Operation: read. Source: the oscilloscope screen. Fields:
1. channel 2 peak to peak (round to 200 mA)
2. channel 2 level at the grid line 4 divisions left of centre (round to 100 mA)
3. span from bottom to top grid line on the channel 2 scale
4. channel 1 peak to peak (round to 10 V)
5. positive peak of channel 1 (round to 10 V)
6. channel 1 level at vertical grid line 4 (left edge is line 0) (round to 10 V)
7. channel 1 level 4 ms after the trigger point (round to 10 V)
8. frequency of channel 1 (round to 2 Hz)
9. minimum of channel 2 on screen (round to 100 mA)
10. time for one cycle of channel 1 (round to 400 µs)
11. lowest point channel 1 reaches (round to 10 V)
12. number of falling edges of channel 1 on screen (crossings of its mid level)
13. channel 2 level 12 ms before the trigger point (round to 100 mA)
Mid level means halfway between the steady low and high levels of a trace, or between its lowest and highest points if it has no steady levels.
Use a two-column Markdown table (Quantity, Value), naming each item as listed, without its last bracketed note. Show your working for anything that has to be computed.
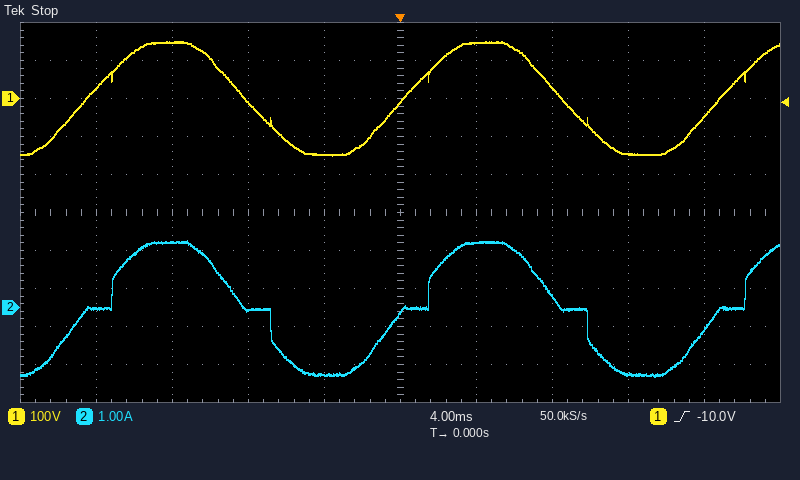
| Quantity | Value |
|---|---|
| channel 2 peak to peak | 3.6 A |
| channel 2 level at the grid line 4 divisions left of centre | 0.0 A |
| span from bottom to top grid line on the channel 2 scale | 10 A |
| channel 1 peak to peak | 150 V − (-150 V) = 300 V |
| positive peak of channel 1 | 150 V |
| channel 1 level at vertical grid line 4 (left edge is line 0) | -150 V |
| channel 1 level 4 ms after the trigger point | 150 V |
| frequency of channel 1 | 1 / 16.8 ms ≈ 60 Hz |
| minimum of channel 2 on screen | -1.8 A |
| time for one cycle of channel 1 | 16.8 ms |
| lowest point channel 1 reaches | -150 V |
| number of falling edges of channel 1 on screen | 2 |
| channel 2 level 12 ms before the trigger point | 1.7 A |
